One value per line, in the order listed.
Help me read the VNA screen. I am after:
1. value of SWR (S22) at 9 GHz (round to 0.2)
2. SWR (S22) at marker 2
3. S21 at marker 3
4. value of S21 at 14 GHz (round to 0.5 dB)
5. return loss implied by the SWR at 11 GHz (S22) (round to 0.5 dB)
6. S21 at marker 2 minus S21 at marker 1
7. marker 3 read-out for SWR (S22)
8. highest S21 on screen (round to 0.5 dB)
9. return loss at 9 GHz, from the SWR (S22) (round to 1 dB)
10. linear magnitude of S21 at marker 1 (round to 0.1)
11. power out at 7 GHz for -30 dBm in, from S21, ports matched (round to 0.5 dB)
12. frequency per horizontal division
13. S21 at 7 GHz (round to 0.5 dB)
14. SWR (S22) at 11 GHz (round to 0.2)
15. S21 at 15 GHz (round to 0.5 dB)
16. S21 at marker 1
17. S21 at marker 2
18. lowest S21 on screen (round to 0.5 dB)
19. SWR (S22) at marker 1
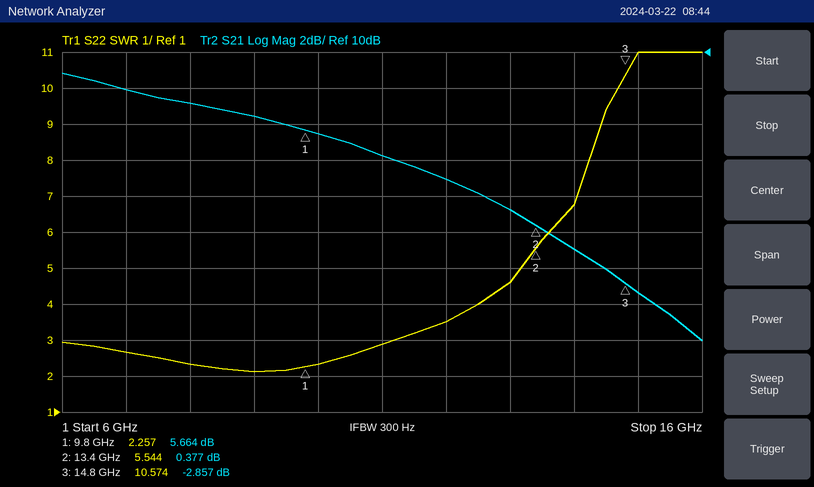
2.2
5.544
-2.857 dB
-1.0 dB
6.5 dB
-5.287 dB
10.574
9.0 dB
9 dB
1.9
-22.0 dBm
1 GHz
8.0 dB
2.8
-3.5 dB
5.664 dB
0.377 dB
-6.0 dB
2.257
